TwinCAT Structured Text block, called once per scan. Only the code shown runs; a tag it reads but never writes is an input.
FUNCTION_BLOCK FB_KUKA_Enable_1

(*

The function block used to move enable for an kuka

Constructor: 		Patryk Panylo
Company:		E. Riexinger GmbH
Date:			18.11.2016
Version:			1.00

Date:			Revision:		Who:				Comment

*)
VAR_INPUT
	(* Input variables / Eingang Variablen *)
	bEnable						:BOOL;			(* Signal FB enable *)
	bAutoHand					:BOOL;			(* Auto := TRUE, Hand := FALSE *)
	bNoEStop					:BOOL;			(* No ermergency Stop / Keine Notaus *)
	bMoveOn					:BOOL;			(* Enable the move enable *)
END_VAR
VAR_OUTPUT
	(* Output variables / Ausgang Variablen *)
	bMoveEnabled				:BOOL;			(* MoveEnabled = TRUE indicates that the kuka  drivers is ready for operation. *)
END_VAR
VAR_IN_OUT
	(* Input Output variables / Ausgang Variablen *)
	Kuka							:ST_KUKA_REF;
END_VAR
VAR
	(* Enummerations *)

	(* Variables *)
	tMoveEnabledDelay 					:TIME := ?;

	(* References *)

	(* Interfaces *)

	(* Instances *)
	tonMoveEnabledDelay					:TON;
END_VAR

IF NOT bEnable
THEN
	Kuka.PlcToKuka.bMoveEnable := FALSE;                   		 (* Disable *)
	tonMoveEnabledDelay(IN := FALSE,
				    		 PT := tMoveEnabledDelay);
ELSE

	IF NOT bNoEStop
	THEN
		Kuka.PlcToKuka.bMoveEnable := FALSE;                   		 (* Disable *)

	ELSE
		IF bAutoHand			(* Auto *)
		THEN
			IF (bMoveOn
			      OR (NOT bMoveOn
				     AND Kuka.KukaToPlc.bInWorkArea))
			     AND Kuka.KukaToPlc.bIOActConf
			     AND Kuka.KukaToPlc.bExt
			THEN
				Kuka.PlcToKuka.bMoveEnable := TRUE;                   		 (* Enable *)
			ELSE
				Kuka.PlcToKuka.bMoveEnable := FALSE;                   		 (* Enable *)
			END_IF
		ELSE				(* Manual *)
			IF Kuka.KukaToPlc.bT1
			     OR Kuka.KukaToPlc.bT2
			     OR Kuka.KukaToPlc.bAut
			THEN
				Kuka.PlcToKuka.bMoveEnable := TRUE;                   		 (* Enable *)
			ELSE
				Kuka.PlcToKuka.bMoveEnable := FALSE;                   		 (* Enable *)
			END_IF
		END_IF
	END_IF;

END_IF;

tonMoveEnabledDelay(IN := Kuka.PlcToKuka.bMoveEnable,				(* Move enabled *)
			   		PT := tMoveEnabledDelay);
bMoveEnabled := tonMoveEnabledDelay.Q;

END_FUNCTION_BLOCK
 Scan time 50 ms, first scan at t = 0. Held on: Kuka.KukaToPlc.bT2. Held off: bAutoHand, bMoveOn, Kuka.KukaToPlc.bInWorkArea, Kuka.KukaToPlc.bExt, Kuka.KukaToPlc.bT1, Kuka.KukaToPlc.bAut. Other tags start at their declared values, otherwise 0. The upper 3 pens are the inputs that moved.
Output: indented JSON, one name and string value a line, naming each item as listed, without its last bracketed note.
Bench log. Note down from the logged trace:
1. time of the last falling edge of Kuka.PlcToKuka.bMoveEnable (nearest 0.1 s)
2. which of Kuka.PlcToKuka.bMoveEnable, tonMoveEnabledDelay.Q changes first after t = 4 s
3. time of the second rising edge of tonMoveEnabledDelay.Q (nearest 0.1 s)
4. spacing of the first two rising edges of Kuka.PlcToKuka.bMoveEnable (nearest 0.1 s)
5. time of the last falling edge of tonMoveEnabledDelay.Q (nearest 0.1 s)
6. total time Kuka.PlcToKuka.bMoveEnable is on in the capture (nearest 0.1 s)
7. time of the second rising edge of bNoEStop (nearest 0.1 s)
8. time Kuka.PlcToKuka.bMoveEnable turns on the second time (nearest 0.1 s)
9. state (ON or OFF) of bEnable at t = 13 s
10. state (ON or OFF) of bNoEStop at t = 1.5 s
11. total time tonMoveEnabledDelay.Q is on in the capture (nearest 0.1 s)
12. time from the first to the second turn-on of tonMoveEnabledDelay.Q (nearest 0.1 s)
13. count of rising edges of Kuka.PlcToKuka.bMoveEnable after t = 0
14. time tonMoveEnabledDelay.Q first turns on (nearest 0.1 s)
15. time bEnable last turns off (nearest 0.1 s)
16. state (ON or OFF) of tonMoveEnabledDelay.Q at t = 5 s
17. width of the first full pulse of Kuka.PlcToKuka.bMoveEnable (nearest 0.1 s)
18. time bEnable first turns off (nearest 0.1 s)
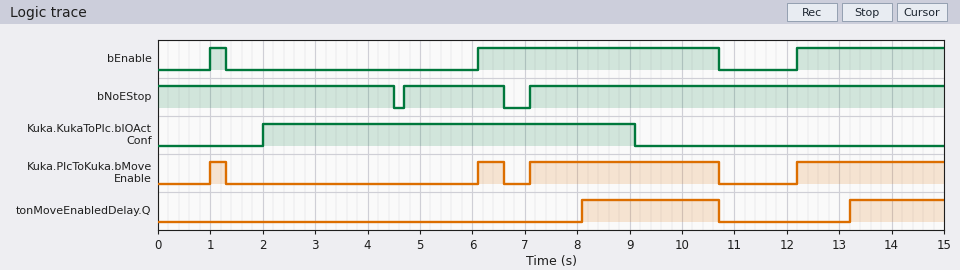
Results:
{
  "time of the last falling edge of Kuka.PlcToKuka.bMoveEnable": "10.7 s",
  "which of Kuka.PlcToKuka.bMoveEnable, tonMoveEnabledDelay.Q changes first after t = 4 s": "Kuka.PlcToKuka.bMoveEnable",
  "time of the second rising edge of tonMoveEnabledDelay.Q": "13.2 s",
  "spacing of the first two rising edges of Kuka.PlcToKuka.bMoveEnable": "5.1 s",
  "time of the last falling edge of tonMoveEnabledDelay.Q": "10.7 s",
  "total time Kuka.PlcToKuka.bMoveEnable is on in the capture": "7.2 s",
  "time of the second rising edge of bNoEStop": "7.1 s",
  "time Kuka.PlcToKuka.bMoveEnable turns on the second time": "6.1 s",
  "state (ON or OFF) of bEnable at t = 13 s": "ON",
  "state (ON or OFF) of bNoEStop at t = 1.5 s": "ON",
  "total time tonMoveEnabledDelay.Q is on in the capture": "4.4 s",
  "time from the first to the second turn-on of tonMoveEnabledDelay.Q": "5.1 s",
  "count of rising edges of Kuka.PlcToKuka.bMoveEnable after t = 0": "4",
  "time tonMoveEnabledDelay.Q first turns on": "8.1 s",
  "time bEnable last turns off": "10.7 s",
  "state (ON or OFF) of tonMoveEnabledDelay.Q at t = 5 s": "OFF",
  "width of the first full pulse of Kuka.PlcToKuka.bMoveEnable": "0.3 s",
  "time bEnable first turns off": "1.3 s"
}
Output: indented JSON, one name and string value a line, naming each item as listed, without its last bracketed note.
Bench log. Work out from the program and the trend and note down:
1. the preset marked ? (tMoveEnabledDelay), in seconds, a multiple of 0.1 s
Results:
{
  "the preset marked ? (tMoveEnabledDelay), in seconds, a multiple of 0.1 s": "1.0 s"
}
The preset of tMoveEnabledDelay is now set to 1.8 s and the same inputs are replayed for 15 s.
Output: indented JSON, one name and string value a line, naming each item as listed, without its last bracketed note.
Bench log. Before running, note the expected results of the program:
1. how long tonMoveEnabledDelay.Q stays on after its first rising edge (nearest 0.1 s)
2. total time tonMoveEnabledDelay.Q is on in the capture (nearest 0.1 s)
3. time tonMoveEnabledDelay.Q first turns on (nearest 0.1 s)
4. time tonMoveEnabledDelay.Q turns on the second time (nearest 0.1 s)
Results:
{
  "how long tonMoveEnabledDelay.Q stays on after its first rising edge": "1.8 s",
  "total time tonMoveEnabledDelay.Q is on in the capture": "2.8 s",
  "time tonMoveEnabledDelay.Q first turns on": "8.9 s",
  "time tonMoveEnabledDelay.Q turns on the second time": "14.0 s"
}
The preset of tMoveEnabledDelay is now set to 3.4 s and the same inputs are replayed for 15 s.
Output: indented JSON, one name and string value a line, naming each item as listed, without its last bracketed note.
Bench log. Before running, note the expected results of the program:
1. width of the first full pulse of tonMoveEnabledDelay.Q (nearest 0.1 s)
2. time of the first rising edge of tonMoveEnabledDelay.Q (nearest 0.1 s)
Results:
{
  "width of the first full pulse of tonMoveEnabledDelay.Q": "0.2 s",
  "time of the first rising edge of tonMoveEnabledDelay.Q": "10.5 s"
}
